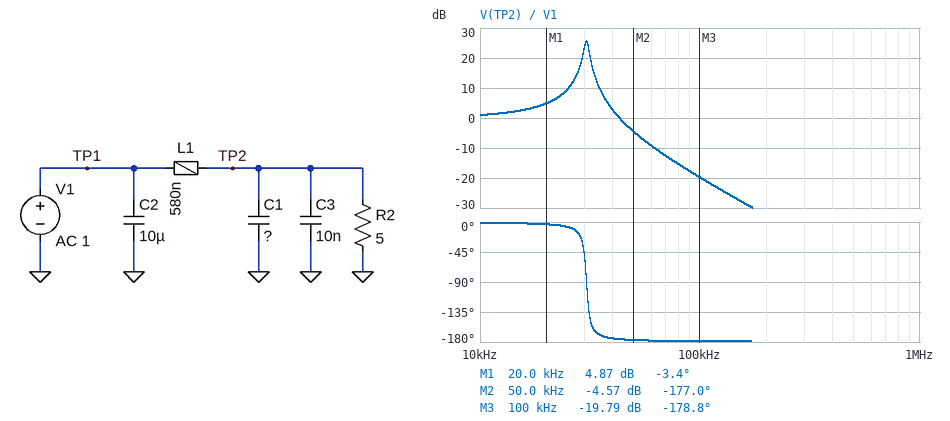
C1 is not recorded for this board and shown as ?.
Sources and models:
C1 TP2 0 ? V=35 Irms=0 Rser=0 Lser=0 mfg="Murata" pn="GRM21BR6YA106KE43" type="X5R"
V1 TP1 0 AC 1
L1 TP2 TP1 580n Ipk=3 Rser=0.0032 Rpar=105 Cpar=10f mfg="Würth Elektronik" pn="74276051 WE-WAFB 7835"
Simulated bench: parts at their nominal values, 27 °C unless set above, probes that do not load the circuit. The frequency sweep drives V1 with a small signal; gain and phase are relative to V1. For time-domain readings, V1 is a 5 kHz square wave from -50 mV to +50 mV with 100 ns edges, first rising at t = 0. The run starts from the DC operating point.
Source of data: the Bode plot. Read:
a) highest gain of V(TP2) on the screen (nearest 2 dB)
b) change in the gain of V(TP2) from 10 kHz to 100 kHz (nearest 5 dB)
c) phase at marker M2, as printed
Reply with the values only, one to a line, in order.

26 dB
-20 dB
-177.0 deg
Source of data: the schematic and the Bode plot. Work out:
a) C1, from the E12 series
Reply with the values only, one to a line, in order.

47 µF
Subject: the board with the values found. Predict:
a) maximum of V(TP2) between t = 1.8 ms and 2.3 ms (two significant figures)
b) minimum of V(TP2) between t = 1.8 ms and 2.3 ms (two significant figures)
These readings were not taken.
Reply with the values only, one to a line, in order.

110 mV
-110 mV
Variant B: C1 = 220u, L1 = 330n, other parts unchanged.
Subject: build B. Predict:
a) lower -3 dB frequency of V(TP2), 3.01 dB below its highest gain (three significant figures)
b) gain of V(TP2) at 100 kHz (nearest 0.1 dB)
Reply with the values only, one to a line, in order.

17.8 kHz
-28.8 dB
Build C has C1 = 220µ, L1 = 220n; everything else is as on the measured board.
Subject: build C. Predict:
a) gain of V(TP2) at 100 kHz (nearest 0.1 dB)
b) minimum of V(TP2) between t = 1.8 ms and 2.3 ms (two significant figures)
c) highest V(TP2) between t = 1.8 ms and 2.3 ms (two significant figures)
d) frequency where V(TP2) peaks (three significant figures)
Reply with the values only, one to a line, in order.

-25.2 dB
-130 mV
130 mV
22.8 kHz
